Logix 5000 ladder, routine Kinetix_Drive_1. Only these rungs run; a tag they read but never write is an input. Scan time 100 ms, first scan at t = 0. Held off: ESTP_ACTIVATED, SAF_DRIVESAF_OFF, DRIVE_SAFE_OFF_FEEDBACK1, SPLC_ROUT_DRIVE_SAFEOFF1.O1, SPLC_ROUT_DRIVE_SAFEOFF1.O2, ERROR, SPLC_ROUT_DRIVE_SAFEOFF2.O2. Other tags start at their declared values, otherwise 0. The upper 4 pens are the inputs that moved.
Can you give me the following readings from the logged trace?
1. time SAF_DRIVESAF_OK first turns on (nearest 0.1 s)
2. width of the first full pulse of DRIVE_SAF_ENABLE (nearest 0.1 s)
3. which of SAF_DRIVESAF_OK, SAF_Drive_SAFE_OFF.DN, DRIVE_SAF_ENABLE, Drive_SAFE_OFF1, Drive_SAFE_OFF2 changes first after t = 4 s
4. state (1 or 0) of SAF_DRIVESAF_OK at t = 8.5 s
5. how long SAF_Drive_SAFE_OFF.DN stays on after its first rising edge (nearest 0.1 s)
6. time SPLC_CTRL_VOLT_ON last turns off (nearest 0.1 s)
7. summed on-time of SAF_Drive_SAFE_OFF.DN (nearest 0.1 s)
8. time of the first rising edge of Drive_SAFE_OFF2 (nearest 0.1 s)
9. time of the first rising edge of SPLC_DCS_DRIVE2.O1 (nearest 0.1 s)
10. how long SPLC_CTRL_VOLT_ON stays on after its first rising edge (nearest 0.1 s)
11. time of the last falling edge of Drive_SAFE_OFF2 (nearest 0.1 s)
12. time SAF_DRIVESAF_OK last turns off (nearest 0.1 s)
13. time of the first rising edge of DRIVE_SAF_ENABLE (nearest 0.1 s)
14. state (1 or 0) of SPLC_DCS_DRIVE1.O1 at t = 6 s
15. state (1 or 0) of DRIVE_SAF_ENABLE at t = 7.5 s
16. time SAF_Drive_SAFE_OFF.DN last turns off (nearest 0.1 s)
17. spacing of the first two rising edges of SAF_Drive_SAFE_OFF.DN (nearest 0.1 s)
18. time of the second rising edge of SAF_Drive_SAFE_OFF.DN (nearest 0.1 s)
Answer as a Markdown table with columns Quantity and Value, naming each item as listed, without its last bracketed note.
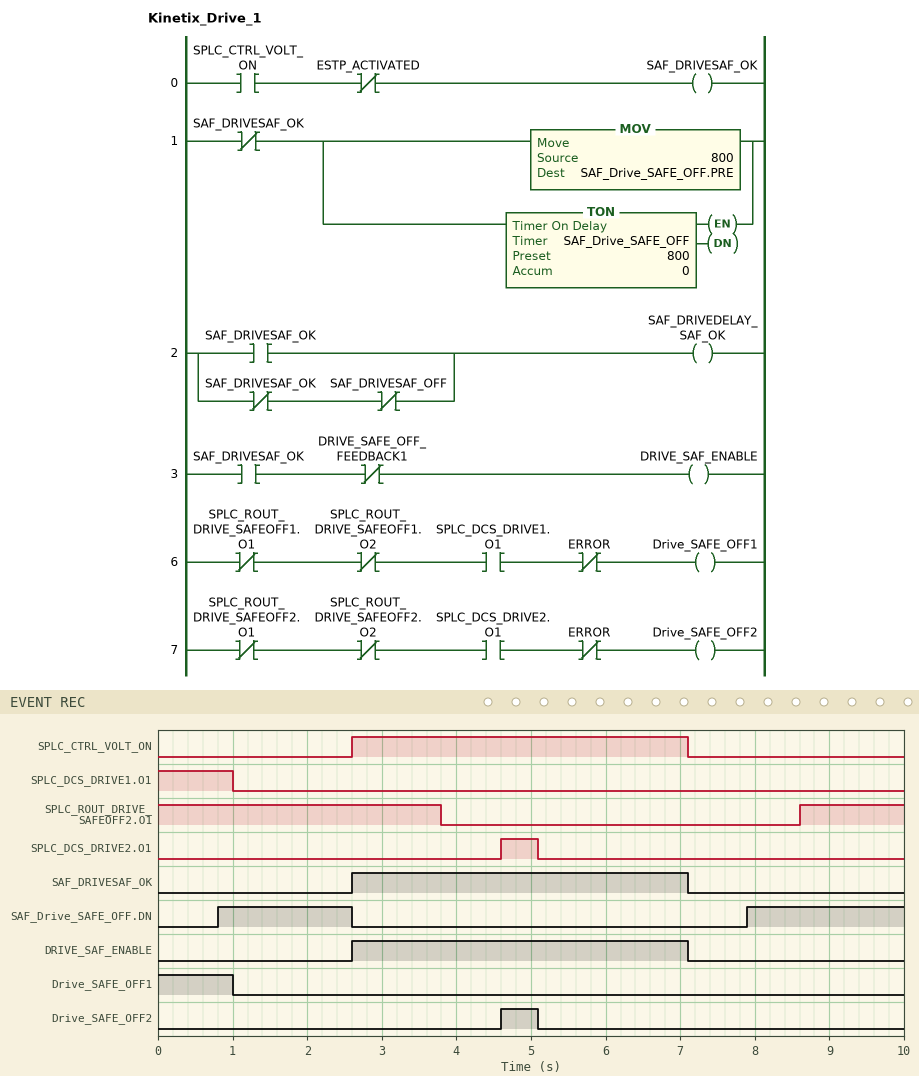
| Quantity | Value |
|---|---|
| time SAF_DRIVESAF_OK first turns on | 2.6 s |
| width of the first full pulse of DRIVE_SAF_ENABLE | 4.5 s |
| which of SAF_DRIVESAF_OK, SAF_Drive_SAFE_OFF.DN, DRIVE_SAF_ENABLE, Drive_SAFE_OFF1, Drive_SAFE_OFF2 changes first after t = 4 s | Drive_SAFE_OFF2 |
| state (1 or 0) of SAF_DRIVESAF_OK at t = 8.5 s | 0 |
| how long SAF_Drive_SAFE_OFF.DN stays on after its first rising edge | 1.8 s |
| time SPLC_CTRL_VOLT_ON last turns off | 7.1 s |
| summed on-time of SAF_Drive_SAFE_OFF.DN | 3.9 s |
| time of the first rising edge of Drive_SAFE_OFF2 | 4.6 s |
| time of the first rising edge of SPLC_DCS_DRIVE2.O1 | 4.6 s |
| how long SPLC_CTRL_VOLT_ON stays on after its first rising edge | 4.5 s |
| time of the last falling edge of Drive_SAFE_OFF2 | 5.1 s |
| time SAF_DRIVESAF_OK last turns off | 7.1 s |
| time of the first rising edge of DRIVE_SAF_ENABLE | 2.6 s |
| state (1 or 0) of SPLC_DCS_DRIVE1.O1 at t = 6 s | 0 |
| state (1 or 0) of DRIVE_SAF_ENABLE at t = 7.5 s | 0 |
| time SAF_Drive_SAFE_OFF.DN last turns off | 2.6 s |
| spacing of the first two rising edges of SAF_Drive_SAFE_OFF.DN | 7.1 s |
| time of the second rising edge of SAF_Drive_SAFE_OFF.DN | 7.9 s |
